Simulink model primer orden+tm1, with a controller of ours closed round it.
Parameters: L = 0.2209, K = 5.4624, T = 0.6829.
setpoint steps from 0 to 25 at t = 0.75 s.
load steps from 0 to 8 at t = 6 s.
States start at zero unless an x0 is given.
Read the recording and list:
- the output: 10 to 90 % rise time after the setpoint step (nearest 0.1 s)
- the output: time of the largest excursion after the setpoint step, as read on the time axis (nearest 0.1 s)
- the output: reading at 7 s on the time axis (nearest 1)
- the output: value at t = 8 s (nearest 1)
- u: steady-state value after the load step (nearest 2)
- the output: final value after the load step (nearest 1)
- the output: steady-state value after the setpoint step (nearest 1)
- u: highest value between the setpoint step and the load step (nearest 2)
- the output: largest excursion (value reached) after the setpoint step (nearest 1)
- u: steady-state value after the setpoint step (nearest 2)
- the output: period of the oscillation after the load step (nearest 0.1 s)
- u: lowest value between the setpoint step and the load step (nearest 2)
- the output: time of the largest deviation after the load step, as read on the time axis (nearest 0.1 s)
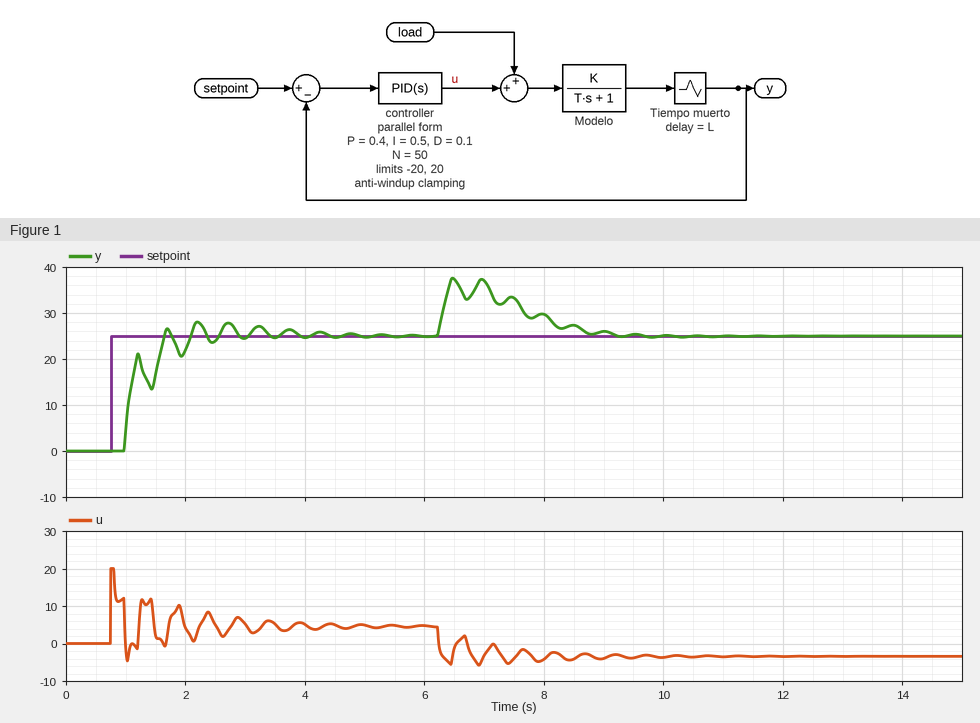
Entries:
0.6 s
2.2 s
37
30
-4
25
25
20
28
4
0.5 s
-4
6.5 s
